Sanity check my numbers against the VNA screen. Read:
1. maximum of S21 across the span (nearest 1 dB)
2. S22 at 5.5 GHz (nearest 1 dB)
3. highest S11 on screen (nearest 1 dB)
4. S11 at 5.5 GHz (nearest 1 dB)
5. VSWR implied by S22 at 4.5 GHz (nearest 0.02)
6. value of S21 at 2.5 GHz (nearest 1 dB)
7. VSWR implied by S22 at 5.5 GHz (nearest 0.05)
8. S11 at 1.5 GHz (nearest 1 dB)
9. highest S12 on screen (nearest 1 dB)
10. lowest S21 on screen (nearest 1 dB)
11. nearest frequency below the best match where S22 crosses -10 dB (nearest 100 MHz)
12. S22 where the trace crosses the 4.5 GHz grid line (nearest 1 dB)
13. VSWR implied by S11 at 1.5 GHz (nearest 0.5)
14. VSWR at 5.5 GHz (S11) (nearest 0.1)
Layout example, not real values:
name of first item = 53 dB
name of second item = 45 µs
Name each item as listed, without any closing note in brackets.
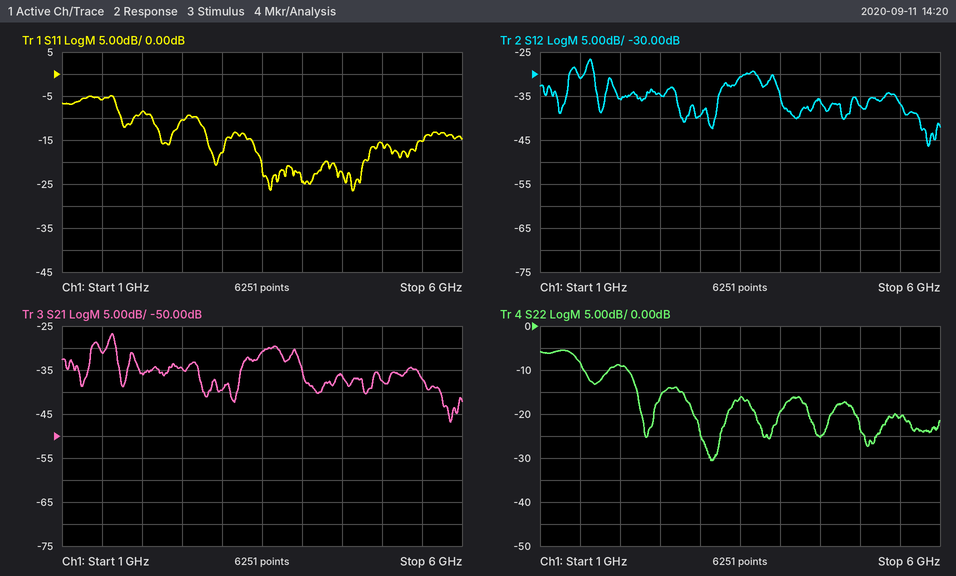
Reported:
maximum of S21 across the span = -27 dB
S22 at 5.5 GHz = -21 dB
highest S11 on screen = -5 dB
S11 at 5.5 GHz = -15 dB
VSWR implied by S22 at 4.5 GHz = 1.12
value of S21 at 2.5 GHz = -35 dB
VSWR implied by S22 at 5.5 GHz = 1.20
S11 at 1.5 GHz = -6 dB
highest S12 on screen = -27 dB
lowest S21 on screen = -47 dB
nearest frequency below the best match where S22 crosses -10 dB = 2.1 GHz
S22 where the trace crosses the 4.5 GHz grid line = -25 dB
VSWR implied by S11 at 1.5 GHz = 3.0
VSWR at 5.5 GHz (S11) = 1.4
